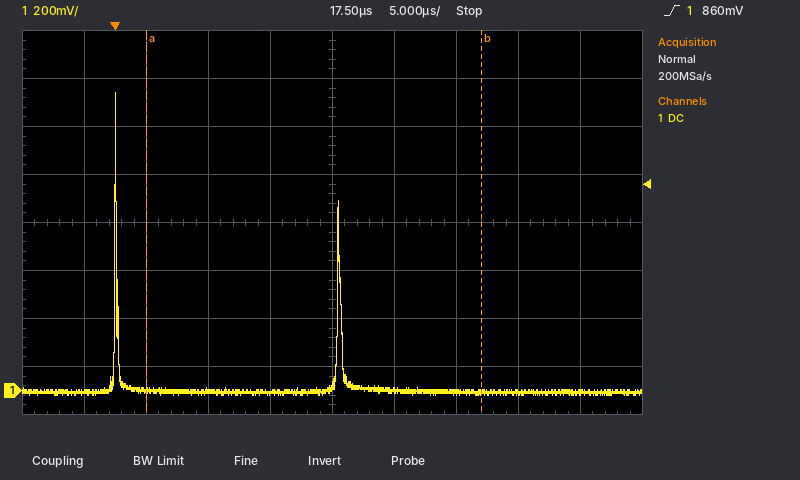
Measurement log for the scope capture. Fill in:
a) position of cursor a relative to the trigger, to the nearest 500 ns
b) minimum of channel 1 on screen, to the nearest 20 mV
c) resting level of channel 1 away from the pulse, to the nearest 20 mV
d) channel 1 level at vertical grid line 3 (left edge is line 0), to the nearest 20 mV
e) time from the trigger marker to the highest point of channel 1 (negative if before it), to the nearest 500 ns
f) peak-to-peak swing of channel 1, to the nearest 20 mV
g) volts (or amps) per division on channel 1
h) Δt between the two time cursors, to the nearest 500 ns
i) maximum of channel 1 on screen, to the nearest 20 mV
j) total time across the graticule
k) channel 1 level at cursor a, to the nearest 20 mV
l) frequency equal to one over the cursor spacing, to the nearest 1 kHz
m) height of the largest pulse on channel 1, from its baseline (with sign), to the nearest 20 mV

+2.5 µs
-20 mV
0 mV
0 mV
0.0 µs
1.26 V
200 mV
27.0 µs
1.24 V
50 µs
0 mV
37 kHz
+1.24 V
